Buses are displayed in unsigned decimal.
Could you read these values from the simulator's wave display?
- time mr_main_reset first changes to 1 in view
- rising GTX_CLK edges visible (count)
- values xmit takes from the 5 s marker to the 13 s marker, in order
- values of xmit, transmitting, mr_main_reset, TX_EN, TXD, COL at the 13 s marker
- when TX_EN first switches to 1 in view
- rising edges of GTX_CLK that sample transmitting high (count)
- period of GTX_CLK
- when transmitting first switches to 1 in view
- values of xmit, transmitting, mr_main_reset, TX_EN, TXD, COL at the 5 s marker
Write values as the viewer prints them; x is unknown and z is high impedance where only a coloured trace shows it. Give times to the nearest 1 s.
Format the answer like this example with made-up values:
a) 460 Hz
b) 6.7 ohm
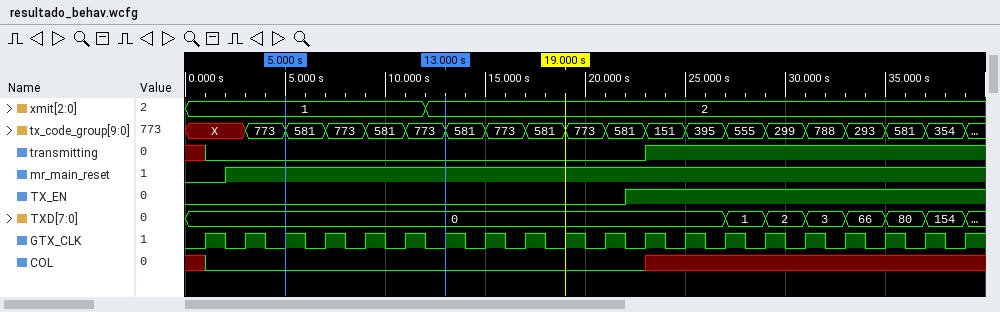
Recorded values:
a) 2 s
b) 20
c) 1, 2
d) xmit=2, transmitting=0, mr_main_reset=1, TX_EN=0, TXD=0, COL=0
e) 22 s
f) 8
g) 2 s
h) 23 s
i) xmit=1, transmitting=0, mr_main_reset=1, TX_EN=0, TXD=0, COL=0
